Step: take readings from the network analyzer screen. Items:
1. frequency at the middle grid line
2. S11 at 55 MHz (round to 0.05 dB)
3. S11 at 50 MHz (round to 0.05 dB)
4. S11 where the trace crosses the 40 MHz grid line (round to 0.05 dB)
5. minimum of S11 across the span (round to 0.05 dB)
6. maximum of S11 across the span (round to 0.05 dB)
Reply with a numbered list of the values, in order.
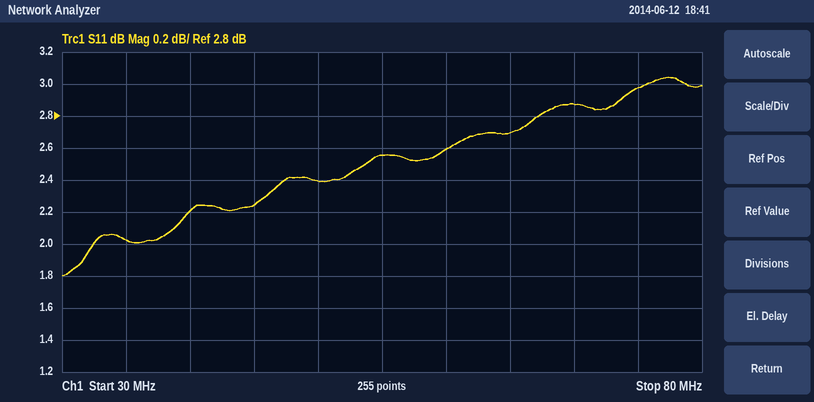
1. 55 MHz
2. 2.55 dB
3. 2.40 dB
4. 2.20 dB
5. 1.80 dB
6. 3.05 dB
